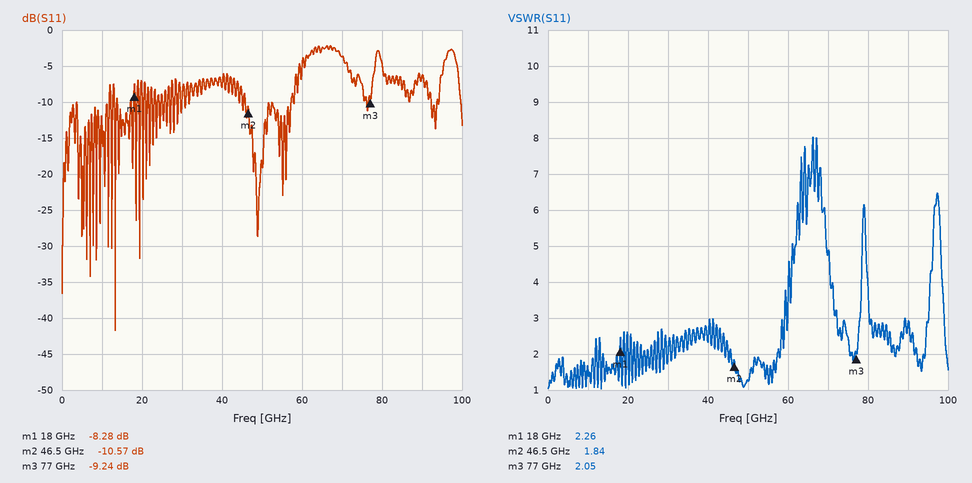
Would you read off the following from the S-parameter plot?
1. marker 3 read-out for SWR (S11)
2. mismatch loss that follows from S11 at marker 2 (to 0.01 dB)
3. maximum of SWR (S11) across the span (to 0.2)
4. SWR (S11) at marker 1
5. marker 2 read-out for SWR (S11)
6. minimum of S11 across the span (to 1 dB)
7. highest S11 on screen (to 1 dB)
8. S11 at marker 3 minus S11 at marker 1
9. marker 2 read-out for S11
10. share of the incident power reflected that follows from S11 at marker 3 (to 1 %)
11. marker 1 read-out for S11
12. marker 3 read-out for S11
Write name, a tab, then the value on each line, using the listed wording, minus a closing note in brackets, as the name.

marker 3 read-out for SWR	2.05
mismatch loss that follows from S11 at marker 2	0.40 dB
maximum of SWR (S11) across the span	8.0
SWR (S11) at marker 1	2.26
marker 2 read-out for SWR	1.84
minimum of S11 across the span	-42 dB
highest S11 on screen	-2 dB
S11 at marker 3 minus S11 at marker 1	-0.96 dB
marker 2 read-out for S11	-10.57 dB
share of the incident power reflected that follows from S11 at marker 3	12 %
marker 1 read-out for S11	-8.28 dB
marker 3 read-out for S11	-9.24 dB
